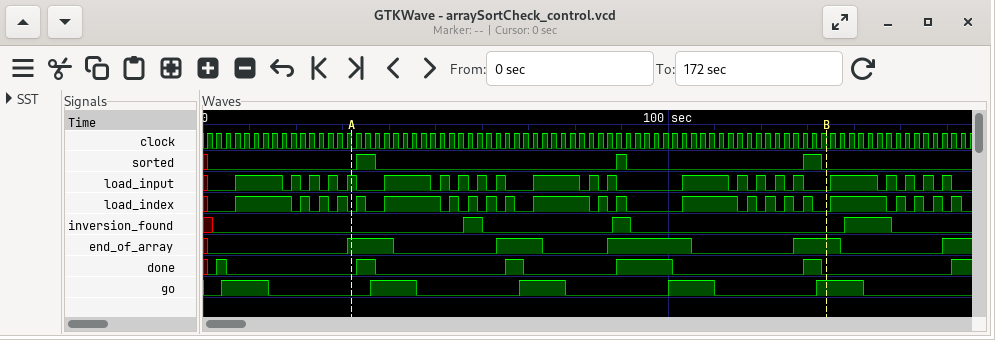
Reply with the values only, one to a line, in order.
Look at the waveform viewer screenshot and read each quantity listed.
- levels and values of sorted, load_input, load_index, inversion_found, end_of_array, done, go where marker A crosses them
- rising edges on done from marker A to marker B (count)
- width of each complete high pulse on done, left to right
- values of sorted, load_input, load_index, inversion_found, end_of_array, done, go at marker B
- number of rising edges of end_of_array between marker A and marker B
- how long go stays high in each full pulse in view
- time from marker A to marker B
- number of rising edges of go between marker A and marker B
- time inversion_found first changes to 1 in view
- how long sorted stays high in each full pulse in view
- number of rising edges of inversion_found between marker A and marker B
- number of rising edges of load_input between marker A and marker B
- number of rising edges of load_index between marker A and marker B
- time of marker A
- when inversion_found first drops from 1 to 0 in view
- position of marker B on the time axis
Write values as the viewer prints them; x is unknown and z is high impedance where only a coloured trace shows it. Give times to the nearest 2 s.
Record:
sorted=0, load_input=1, load_index=0, inversion_found=0, end_of_array=1, done=0, go=0
4
2 s, 4 s, 4 s, 12 s, 4 s
sorted=0, load_input=0, load_index=0, inversion_found=0, end_of_array=1, done=0, go=1
3
10 s, 10 s, 10 s, 10 s, 10 s
102 s
4
56 s
4 s, 2 s, 4 s
2
13
14
32 s
60 s
134 s
